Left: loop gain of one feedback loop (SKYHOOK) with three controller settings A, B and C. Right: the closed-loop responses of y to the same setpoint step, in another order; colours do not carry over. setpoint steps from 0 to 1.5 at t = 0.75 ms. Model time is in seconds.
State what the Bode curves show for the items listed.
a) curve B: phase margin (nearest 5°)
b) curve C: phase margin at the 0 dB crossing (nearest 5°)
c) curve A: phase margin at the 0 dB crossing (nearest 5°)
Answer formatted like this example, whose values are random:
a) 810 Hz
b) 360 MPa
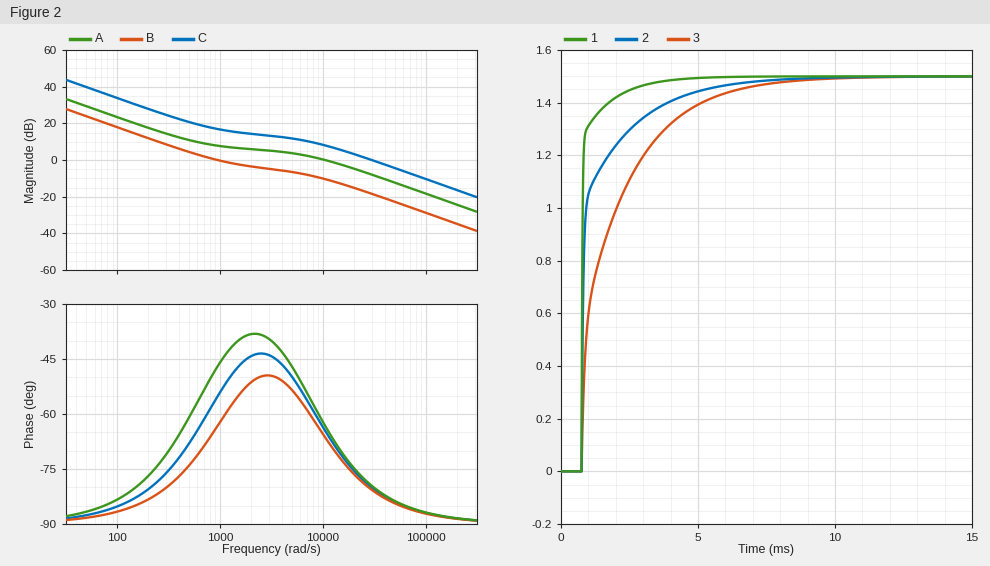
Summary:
a) 115°
b) 100°
c) 115°
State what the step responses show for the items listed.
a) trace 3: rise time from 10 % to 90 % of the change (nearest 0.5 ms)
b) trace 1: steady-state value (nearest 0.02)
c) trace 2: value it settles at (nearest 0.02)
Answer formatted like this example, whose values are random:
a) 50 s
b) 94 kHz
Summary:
a) 3.5 ms
b) 1.50
c) 1.50
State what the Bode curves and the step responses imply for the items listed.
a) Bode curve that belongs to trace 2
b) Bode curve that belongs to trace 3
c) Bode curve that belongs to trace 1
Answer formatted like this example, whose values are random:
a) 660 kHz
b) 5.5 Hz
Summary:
a) A
b) B
c) C
